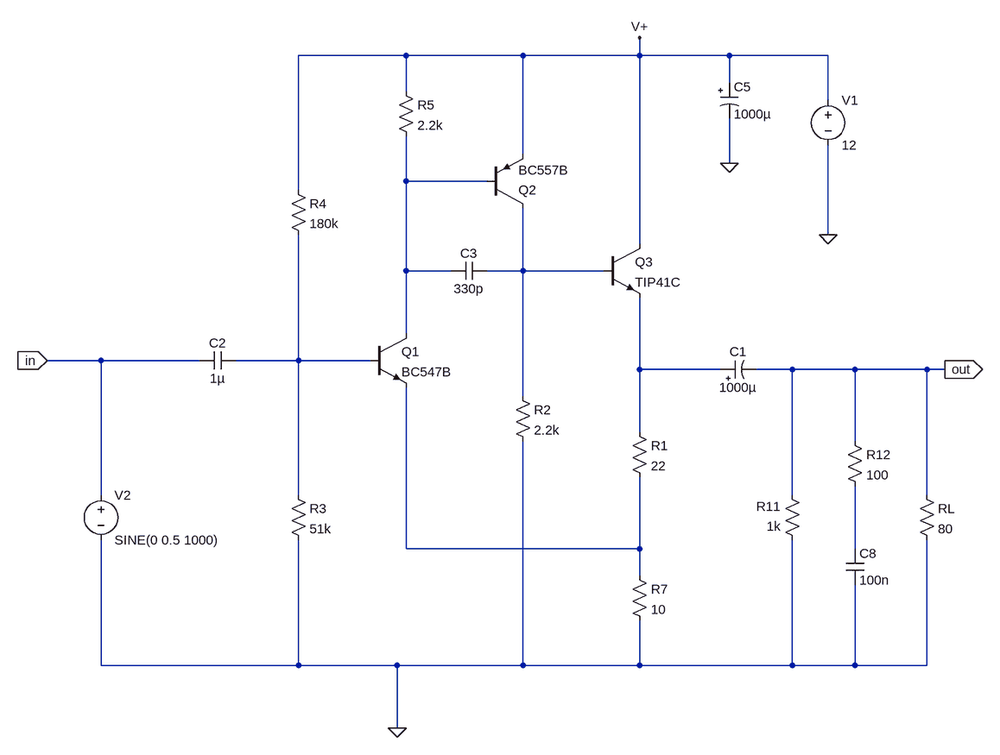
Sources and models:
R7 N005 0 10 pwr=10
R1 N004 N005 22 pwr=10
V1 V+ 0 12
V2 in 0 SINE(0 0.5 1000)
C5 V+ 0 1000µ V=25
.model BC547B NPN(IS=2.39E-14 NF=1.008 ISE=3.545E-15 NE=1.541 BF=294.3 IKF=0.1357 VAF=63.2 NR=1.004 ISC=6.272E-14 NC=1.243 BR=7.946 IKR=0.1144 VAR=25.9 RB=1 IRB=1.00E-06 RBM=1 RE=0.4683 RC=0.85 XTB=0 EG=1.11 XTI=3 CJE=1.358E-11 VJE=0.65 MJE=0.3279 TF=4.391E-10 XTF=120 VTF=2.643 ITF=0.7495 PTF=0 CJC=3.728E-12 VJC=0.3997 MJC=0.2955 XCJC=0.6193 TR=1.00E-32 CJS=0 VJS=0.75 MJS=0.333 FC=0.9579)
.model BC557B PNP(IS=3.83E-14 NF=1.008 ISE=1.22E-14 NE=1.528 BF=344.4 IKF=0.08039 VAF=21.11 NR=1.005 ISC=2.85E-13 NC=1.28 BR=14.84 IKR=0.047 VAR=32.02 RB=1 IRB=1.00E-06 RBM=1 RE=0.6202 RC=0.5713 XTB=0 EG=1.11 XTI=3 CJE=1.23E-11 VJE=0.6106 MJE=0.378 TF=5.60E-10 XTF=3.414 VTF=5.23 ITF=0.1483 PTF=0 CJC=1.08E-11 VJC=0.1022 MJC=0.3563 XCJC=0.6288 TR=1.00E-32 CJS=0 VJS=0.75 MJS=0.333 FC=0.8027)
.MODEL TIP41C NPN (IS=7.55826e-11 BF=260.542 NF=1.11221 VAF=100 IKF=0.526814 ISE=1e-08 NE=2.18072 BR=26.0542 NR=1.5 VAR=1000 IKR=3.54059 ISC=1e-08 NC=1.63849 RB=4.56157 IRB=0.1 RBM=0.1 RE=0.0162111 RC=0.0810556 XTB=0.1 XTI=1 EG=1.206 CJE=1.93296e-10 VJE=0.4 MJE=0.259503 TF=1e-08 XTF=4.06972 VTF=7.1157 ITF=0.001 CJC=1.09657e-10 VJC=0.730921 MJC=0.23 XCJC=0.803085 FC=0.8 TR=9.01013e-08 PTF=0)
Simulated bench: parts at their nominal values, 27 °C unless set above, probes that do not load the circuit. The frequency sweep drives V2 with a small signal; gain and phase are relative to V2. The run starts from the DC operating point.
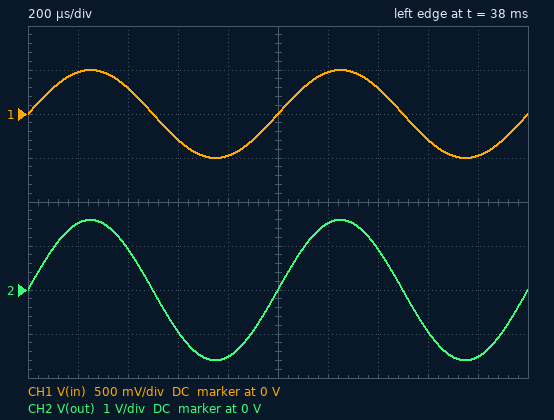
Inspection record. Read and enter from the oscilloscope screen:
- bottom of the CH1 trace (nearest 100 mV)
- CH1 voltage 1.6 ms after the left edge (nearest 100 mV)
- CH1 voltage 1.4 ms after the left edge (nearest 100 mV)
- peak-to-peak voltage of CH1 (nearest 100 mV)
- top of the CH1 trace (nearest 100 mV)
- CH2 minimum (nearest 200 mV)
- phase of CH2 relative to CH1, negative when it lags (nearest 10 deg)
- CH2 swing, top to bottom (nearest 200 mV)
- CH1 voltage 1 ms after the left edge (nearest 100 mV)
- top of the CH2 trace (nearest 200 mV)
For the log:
-500 mV
-300 mV
300 mV
1.0 V
500 mV
-1.6 V
0 deg
3.2 V
0 V
1.6 V
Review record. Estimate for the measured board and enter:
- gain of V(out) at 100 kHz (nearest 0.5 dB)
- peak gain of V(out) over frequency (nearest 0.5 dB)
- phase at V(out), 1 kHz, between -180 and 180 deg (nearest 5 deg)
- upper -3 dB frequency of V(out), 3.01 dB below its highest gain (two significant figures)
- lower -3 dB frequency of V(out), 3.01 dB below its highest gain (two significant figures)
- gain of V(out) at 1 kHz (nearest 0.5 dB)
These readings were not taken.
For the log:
10.0 dB
10.0 dB
0 deg
1.8 MHz
4.9 Hz
10.0 dB
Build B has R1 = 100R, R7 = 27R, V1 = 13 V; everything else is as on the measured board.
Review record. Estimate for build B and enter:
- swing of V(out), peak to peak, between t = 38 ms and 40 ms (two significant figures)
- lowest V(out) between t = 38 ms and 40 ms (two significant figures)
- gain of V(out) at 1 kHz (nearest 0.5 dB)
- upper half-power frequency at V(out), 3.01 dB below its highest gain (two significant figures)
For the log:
4.3 V
-2.4 V
13.5 dB
1.0 MHz
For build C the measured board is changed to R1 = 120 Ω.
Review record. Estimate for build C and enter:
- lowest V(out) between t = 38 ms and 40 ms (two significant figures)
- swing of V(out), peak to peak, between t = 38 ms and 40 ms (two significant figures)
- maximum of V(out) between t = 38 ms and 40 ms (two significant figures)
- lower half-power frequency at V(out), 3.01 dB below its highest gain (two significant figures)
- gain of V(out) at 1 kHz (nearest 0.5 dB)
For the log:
-3.9 V
4.6 V
750 mV
45 Hz
-29.0 dB
